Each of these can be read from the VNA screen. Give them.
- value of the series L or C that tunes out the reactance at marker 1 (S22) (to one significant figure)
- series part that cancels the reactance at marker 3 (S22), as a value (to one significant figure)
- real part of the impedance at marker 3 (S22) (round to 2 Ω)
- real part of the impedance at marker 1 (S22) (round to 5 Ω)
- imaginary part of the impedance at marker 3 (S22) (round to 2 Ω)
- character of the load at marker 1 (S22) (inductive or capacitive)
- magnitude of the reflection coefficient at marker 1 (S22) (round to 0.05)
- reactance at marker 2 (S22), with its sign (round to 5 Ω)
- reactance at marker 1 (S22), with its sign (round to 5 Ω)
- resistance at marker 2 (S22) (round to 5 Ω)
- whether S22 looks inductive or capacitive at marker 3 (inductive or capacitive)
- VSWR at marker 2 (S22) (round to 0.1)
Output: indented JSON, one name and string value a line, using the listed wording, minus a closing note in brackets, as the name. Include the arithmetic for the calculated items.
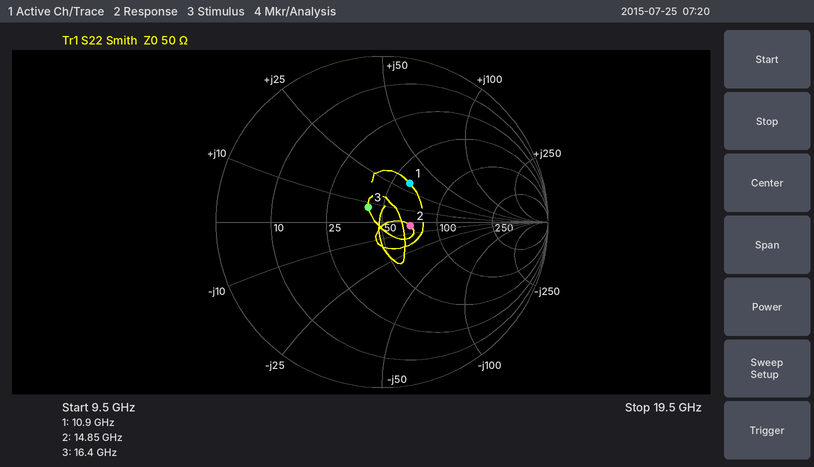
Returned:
{
  "value of the series L or C that tunes out the reactance at marker 1 (S22)": "C = 1/(2π × 10.9 GHz × 30 Ω) ≈ 487 fF, so 500 fF to one significant figure",
  "series part that cancels the reactance at marker 3 (S22), as a value": "C = 1/(2π × 16.4 GHz × 8 Ω) ≈ 1 pF",
  "real part of the impedance at marker 3 (S22)": "42 Ω",
  "real part of the impedance at marker 1 (S22)": "60 Ω",
  "imaginary part of the impedance at marker 3 (S22)": "+8 Ω",
  "character of the load at marker 1 (S22)": "inductive",
  "magnitude of the reflection coefficient at marker 1 (S22)": "0.30",
  "reactance at marker 2 (S22), with its sign": "-5 Ω",
  "reactance at marker 1 (S22), with its sign": "+30 Ω",
  "resistance at marker 2 (S22)": "70 Ω",
  "whether S22 looks inductive or capacitive at marker 3": "inductive",
  "VSWR at marker 2 (S22)": "1.4"
}
